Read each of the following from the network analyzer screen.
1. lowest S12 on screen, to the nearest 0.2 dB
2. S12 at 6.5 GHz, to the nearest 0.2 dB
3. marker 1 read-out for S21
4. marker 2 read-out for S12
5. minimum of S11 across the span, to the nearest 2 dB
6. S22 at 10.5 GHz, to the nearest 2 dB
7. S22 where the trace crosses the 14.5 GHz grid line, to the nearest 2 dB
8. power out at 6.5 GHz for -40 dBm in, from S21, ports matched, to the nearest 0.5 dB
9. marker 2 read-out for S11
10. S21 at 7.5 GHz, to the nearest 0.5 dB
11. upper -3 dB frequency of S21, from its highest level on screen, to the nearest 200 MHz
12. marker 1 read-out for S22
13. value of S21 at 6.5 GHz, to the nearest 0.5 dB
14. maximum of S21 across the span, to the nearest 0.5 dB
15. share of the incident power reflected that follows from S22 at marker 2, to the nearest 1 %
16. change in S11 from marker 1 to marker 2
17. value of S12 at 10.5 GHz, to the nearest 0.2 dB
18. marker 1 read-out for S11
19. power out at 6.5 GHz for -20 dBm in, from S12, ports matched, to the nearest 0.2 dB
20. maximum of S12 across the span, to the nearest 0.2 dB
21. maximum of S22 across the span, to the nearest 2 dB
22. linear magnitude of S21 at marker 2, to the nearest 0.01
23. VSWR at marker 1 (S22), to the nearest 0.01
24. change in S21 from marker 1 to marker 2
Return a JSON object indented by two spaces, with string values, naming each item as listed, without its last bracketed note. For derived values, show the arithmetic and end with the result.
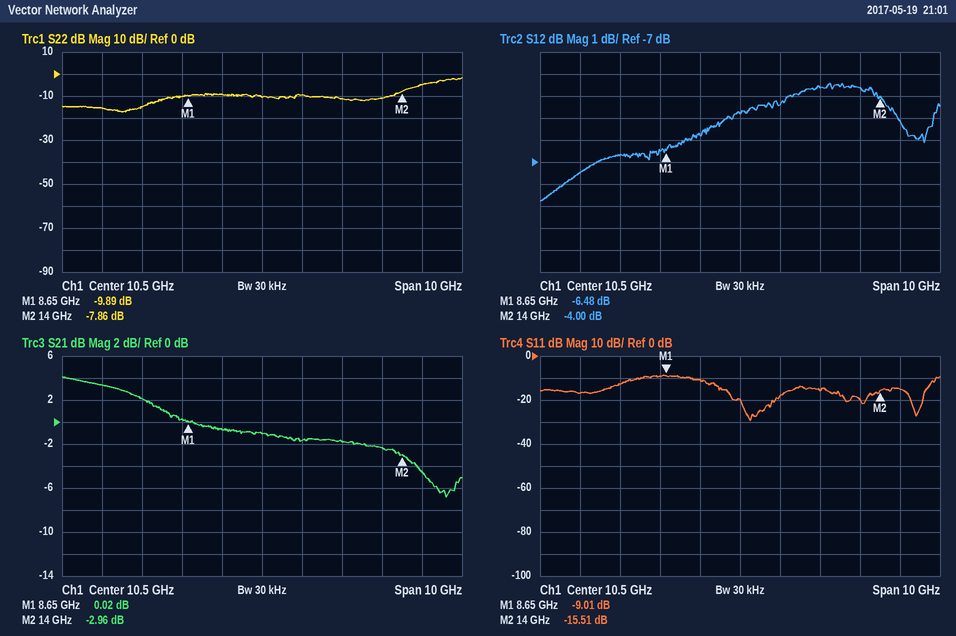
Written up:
{
  "lowest S12 on screen, to the nearest 0.2 dB": "-8.8 dB",
  "S12 at 6.5 GHz, to the nearest 0.2 dB": "-7.4 dB",
  "marker 1 read-out for S21": "0.02 dB",
  "marker 2 read-out for S12": "-4.00 dB",
  "minimum of S11 across the span, to the nearest 2 dB": "-30 dB",
  "S22 at 10.5 GHz, to the nearest 2 dB": "-10 dB",
  "S22 where the trace crosses the 14.5 GHz grid line, to the nearest 2 dB": "-4 dB",
  "power out at 6.5 GHz for -40 dBm in, from S21, ports matched, to the nearest 0.5 dB": "-40 dBm + (3.5 dB) = -36.5 dBm",
  "marker 2 read-out for S11": "-15.51 dB",
  "S21 at 7.5 GHz, to the nearest 0.5 dB": "2.0 dB",
  "upper -3 dB frequency of S21, from its highest level on screen, to the nearest 200 MHz": "8.0 GHz",
  "marker 1 read-out for S22": "-9.89 dB",
  "value of S21 at 6.5 GHz, to the nearest 0.5 dB": "3.5 dB",
  "maximum of S21 across the span, to the nearest 0.5 dB": "4.0 dB",
  "share of the incident power reflected that follows from S22 at marker 2, to the nearest 1 %": "10^(-7.86/10) ≈ 16 %",
  "change in S11 from marker 1 to marker 2": "-15.51 − (-9.01) = -6.50 dB",
  "value of S12 at 10.5 GHz, to the nearest 0.2 dB": "-4.8 dB",
  "marker 1 read-out for S11": "-9.01 dB",
  "power out at 6.5 GHz for -20 dBm in, from S12, ports matched, to the nearest 0.2 dB": "-20 dBm + (-7.4 dB) = -27.4 dBm",
  "maximum of S12 across the span, to the nearest 0.2 dB": "-3.4 dB",
  "maximum of S22 across the span, to the nearest 2 dB": "-2 dB",
  "linear magnitude of S21 at marker 2, to the nearest 0.01": "10^(-2.96/20) ≈ 0.71",
  "VSWR at marker 1 (S22), to the nearest 0.01": "(1 + 0.3203)/(1 − 0.3203) ≈ 1.94",
  "change in S21 from marker 1 to marker 2": "-2.96 − (0.02) = -2.98 dB"
}
